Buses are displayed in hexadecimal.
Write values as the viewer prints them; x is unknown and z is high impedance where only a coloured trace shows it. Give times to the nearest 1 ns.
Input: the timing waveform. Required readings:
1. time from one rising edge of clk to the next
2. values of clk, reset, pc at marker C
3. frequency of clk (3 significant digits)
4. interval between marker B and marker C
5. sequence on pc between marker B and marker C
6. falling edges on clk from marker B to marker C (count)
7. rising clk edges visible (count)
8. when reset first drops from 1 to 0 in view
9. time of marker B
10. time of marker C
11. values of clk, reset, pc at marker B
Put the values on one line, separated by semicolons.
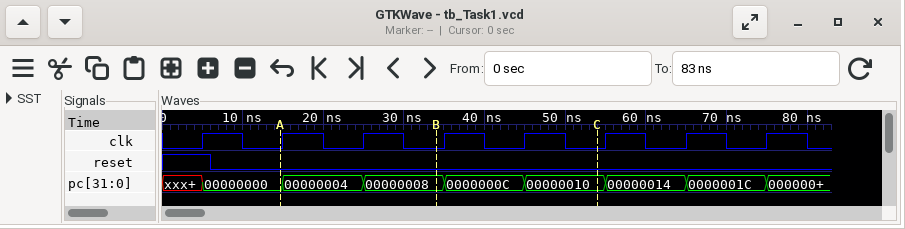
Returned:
10 ns; clk=0, reset=0, pc=00000010; 100 MHz; 20 ns; 00000008, 0000000C, 00000010; 2; 8; 6 ns; 34 ns; 54 ns; clk=0, reset=0, pc=00000008
